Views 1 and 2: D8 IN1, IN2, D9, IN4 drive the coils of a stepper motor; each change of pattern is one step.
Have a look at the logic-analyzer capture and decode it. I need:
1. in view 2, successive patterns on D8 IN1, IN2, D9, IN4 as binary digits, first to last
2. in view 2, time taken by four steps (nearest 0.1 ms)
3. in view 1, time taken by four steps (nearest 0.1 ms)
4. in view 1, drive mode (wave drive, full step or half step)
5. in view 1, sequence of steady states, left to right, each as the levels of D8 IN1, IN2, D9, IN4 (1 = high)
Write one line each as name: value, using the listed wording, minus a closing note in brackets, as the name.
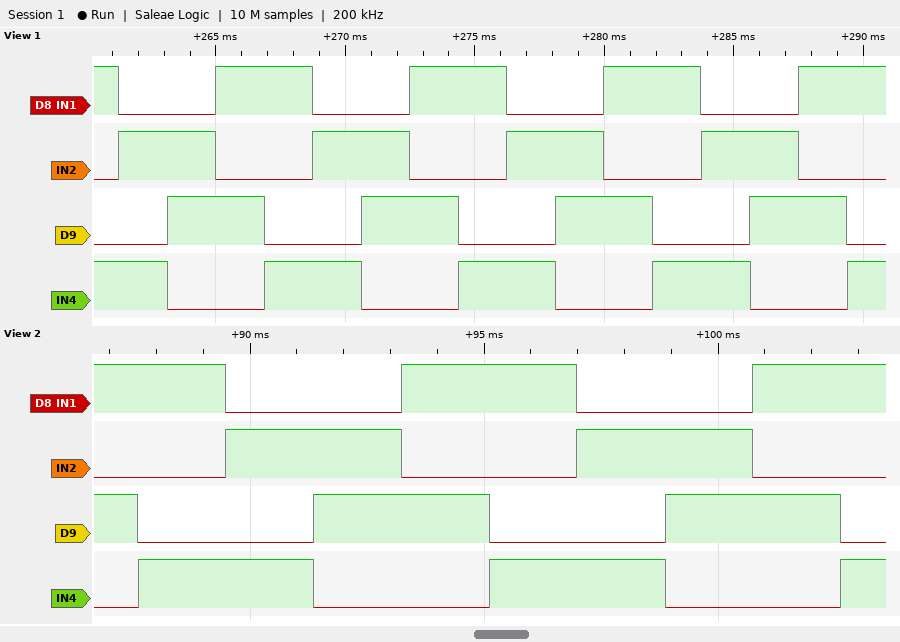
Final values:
in view 2, successive patterns on D8 IN1, IN2, D9, IN4 as binary digits, first to last: 1010 1001 0101 0110 1010 1001 0101 0110 1010 1001
in view 2, time taken by four steps: 7.5 ms
in view 1, time taken by four steps: 7.5 ms
in view 1, drive mode: full step
in view 1, sequence of steady states, left to right, each as the levels of D8 IN1, IN2, D9, IN4: 1001 0101 0110 1010 1001 0101 0110 1010 1001 0101 0110 1010 1001 0101 0110 1010 1001
